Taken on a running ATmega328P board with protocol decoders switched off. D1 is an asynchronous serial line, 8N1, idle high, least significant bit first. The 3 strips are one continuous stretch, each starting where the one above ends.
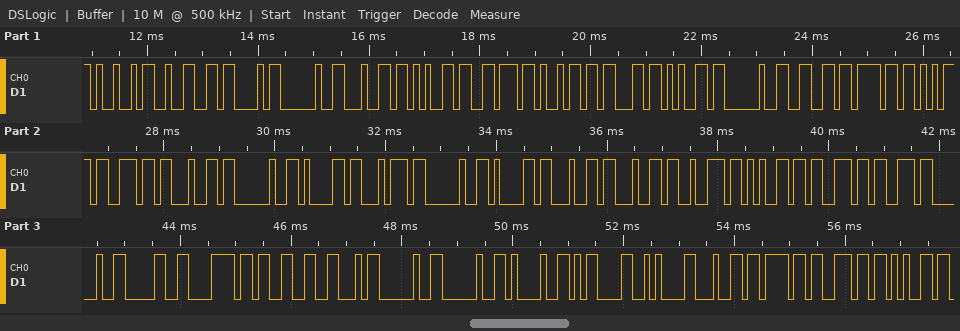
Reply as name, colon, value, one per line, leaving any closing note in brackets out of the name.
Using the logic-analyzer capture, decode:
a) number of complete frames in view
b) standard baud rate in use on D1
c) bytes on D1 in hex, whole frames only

number of complete frames in view: 41
standard baud rate in use on D1: 9600 baud
bytes on D1 in hex, whole frames only: 49 32 43 20 64 65 76 69 63 65 20 66 6F 75 6E 64 20 61 74 20 61 64 64 72 65 73 73 20 30 78 33 46 20 20 21 0D 0A 64 6F 6E 65
